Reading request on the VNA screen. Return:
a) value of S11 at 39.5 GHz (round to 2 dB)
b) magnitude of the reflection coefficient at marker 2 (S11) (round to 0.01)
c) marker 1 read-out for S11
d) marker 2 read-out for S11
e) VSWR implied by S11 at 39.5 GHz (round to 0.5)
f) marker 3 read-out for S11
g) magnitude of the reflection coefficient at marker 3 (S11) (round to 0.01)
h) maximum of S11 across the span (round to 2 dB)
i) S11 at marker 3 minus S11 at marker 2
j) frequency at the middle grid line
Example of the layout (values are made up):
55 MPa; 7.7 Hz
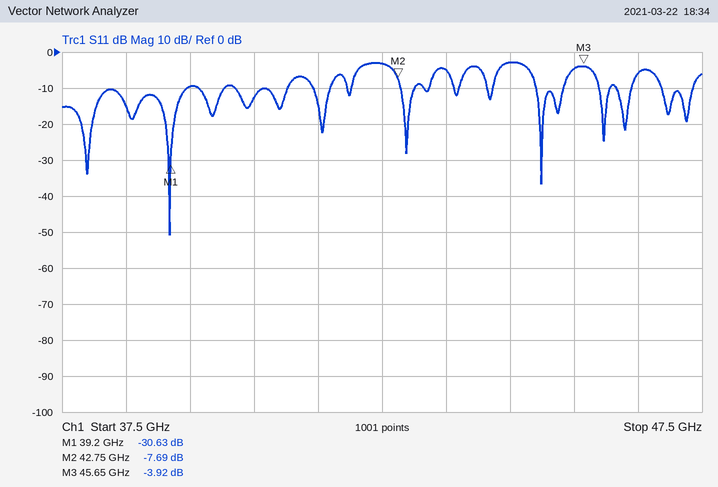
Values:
-10 dB; 0.41; -30.63 dB; -7.69 dB; 2.0; -3.92 dB; 0.64; -2 dB; 3.77 dB; 42.5 GHz
